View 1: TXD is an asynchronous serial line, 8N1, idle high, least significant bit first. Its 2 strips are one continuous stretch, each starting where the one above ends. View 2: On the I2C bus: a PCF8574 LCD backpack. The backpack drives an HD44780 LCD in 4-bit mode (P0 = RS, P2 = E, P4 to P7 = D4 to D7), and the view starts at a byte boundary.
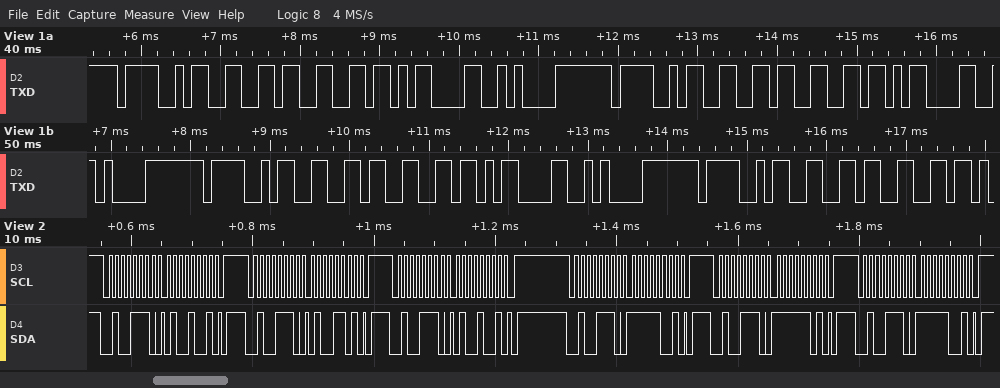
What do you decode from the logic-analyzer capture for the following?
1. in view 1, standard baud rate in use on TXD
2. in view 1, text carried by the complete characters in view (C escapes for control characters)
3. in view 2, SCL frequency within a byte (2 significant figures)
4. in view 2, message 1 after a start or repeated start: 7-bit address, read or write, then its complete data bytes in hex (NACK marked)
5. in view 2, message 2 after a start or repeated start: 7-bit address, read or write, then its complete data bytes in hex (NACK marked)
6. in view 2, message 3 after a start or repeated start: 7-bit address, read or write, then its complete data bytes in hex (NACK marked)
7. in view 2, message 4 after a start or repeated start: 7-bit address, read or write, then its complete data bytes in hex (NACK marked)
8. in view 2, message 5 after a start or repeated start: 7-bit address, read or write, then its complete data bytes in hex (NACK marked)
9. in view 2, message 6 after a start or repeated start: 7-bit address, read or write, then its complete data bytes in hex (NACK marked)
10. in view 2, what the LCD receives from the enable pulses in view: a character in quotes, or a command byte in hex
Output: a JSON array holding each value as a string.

["9600 baud", "\"Off\\r\\nOff\\r\\nOff\\r\\nOff\"", "100 kHz", "0x27 write: 49", "0x27 write: 4D", "0x27 write: 49", "0x27 write: F9", "0x27 write: FD", "0x27 write: F9", "'O'"]
